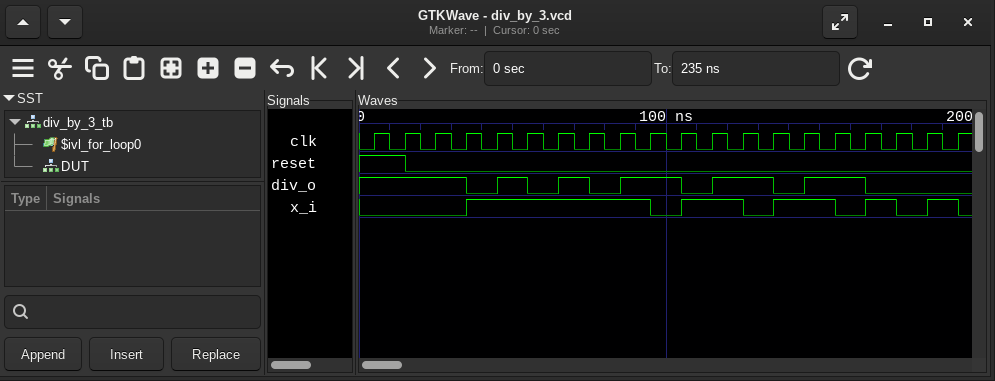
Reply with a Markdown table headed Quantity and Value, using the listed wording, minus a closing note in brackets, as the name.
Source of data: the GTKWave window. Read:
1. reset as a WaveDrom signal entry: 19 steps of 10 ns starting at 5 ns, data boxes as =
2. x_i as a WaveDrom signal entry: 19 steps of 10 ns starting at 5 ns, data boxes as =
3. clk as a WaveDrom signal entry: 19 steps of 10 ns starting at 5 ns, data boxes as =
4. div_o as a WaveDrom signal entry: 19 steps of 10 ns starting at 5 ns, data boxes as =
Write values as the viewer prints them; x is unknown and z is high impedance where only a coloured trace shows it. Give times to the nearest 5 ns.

| Quantity | Value |
|---|---|
| reset as a WaveDrom signal entry: 19 steps of 10 ns starting at 5 ns, data boxes as = | {name: 'reset', wave: '10.................'} |
| x_i as a WaveDrom signal entry: 19 steps of 10 ns starting at 5 ns, data boxes as = | {name: 'x_i', wave: '0..1.....01.01.0101'} |
| clk as a WaveDrom signal entry: 19 steps of 10 ns starting at 5 ns, data boxes as = | {name: 'clk', wave: 'p..................'} |
| div_o as a WaveDrom signal entry: 19 steps of 10 ns starting at 5 ns, data boxes as = | {name: 'div_o', wave: '1..010101.01.01.0..'} |
